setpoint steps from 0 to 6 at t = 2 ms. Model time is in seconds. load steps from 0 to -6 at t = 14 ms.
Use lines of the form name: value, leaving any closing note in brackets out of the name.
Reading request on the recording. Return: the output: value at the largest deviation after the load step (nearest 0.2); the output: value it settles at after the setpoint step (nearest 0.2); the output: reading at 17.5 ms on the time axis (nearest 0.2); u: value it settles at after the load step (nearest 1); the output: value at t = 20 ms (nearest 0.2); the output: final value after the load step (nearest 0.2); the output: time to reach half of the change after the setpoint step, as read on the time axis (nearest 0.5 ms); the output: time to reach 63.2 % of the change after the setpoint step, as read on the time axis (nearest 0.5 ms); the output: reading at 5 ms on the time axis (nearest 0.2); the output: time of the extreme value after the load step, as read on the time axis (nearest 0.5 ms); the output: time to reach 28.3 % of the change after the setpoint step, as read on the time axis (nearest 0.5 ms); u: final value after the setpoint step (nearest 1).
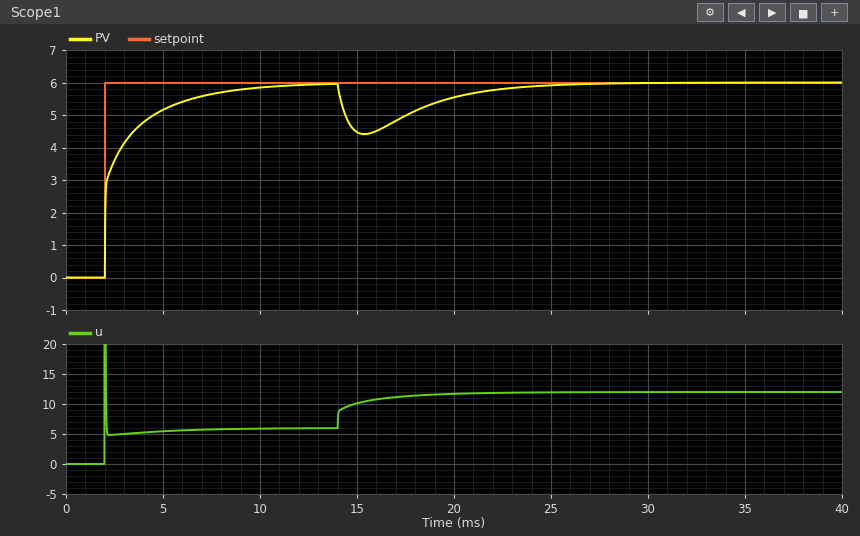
the output: value at the largest deviation after the load step: 4.4
the output: value it settles at after the setpoint step: 6.0
the output: reading at 17.5 ms on the time axis: 5.0
u: value it settles at after the load step: 12
the output: value at t = 20 ms: 5.6
the output: final value after the load step: 6.0
the output: time to reach half of the change after the setpoint step, as read on the time axis: 2.0 ms
the output: time to reach 63.2 % of the change after the setpoint step, as read on the time axis: 2.5 ms
the output: reading at 5 ms on the time axis: 5.2
the output: time of the extreme value after the load step, as read on the time axis: 15.5 ms
the output: time to reach 28.3 % of the change after the setpoint step, as read on the time axis: 2.0 ms
u: final value after the setpoint step: 6
